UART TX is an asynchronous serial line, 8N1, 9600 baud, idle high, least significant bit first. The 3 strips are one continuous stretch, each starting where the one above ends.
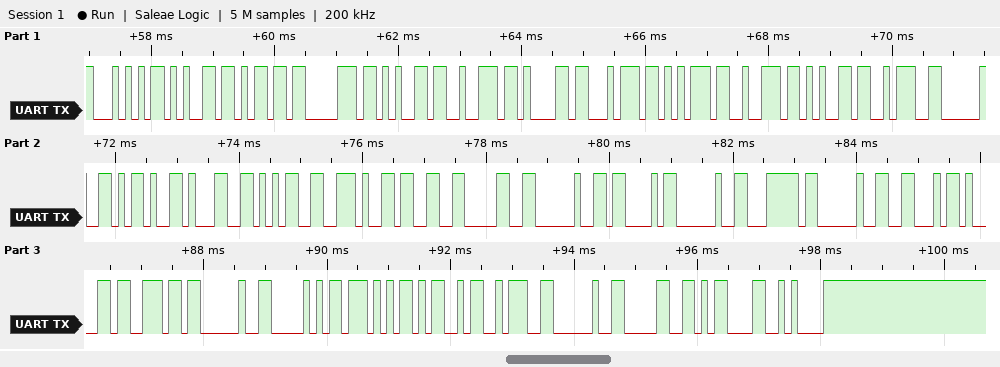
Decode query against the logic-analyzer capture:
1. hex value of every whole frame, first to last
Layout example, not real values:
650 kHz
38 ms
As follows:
54 65 6D 70 65 72 61 74 75 72 65 3A 20 2D 31 35 2E 33 30 20 43 20 7C 20 46 61 6E 20 50 57 4D 3A 20 30 0D 0A
